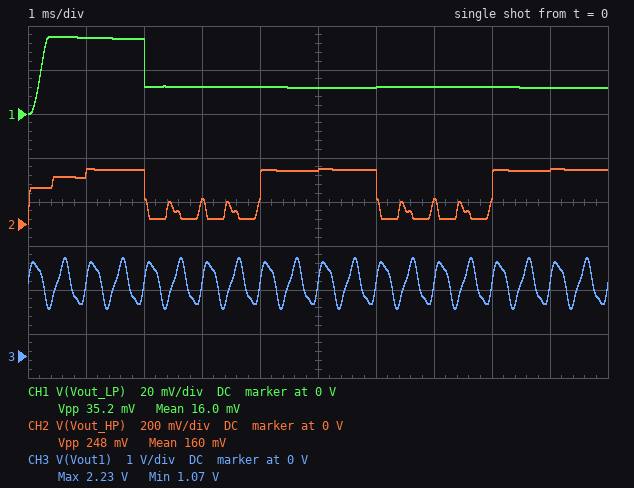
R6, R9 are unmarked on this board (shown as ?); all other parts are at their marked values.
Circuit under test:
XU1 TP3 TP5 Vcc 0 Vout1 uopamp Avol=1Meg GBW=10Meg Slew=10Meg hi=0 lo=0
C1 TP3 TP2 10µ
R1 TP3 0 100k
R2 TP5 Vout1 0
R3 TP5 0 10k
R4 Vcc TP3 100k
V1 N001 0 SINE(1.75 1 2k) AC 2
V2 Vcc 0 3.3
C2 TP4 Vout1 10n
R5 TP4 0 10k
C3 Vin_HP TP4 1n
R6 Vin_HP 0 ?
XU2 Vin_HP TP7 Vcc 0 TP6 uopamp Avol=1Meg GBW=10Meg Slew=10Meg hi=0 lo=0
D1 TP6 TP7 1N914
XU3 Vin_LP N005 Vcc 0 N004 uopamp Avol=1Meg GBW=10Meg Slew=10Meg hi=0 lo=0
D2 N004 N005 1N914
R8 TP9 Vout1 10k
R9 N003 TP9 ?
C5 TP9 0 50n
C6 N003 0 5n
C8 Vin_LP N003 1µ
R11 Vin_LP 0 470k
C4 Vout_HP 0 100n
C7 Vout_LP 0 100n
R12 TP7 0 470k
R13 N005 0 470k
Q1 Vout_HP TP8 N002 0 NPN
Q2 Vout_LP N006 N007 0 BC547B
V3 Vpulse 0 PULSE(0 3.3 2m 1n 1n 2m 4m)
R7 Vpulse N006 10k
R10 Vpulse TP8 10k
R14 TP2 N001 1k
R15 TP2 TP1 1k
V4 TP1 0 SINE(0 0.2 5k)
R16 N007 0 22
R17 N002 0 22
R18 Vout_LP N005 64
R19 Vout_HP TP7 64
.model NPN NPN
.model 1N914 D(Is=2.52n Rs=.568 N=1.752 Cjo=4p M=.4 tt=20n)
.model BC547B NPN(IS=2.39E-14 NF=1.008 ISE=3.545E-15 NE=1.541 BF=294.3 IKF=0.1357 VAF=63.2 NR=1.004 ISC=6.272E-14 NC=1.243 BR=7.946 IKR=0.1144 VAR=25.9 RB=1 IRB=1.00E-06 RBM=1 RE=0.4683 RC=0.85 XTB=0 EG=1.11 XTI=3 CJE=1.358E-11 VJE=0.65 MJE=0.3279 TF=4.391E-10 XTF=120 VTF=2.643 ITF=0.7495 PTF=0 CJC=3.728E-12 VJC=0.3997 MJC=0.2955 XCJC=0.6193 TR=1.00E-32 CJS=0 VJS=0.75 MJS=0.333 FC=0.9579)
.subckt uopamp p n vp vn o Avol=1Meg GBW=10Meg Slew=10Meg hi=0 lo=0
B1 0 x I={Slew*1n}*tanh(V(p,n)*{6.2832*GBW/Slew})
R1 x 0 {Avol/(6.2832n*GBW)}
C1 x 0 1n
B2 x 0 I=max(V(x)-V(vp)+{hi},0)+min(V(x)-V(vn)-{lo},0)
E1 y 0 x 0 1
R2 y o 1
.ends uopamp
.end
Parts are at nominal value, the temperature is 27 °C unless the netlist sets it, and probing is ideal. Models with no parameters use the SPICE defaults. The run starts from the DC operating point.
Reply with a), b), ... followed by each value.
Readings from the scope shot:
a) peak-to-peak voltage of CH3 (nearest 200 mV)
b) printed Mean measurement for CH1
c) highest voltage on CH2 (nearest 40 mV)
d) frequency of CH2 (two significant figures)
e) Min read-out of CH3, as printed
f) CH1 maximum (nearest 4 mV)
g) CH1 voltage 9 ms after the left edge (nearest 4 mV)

a) 1.2 V
b) 16.0 mV
c) 240 mV
d) 250 Hz
e) 1.07 V
f) 36 mV
g) 12 mV
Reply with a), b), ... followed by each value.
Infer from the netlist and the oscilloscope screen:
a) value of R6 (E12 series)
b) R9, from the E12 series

a) 47 kΩ
b) 120 kΩ
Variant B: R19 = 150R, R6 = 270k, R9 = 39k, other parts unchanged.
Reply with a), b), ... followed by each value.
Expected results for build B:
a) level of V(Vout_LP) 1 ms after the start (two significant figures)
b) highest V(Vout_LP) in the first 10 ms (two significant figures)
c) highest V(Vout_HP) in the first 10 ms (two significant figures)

a) 71 mV
b) 72 mV
c) 450 mV
